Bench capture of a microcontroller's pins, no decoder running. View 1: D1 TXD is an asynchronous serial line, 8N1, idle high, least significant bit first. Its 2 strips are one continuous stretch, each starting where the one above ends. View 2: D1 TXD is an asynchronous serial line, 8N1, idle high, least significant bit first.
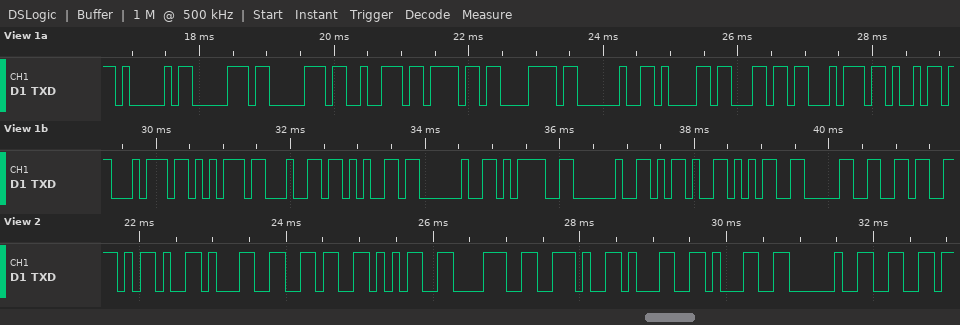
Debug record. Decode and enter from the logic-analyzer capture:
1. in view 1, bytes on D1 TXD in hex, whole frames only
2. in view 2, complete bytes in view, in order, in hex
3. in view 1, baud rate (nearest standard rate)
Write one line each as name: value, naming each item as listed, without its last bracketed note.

in view 1, bytes on D1 TXD in hex, whole frames only: 0x41 0x70 0x70 0x72 0x6F 0x78 0x20 0x61 0x6C 0x74 0x69 0x74 0x75 0x64 0x65 0x20 0x3D 0x20 0x2D 0x35 0x30 0x36
in view 2, complete bytes in view, in order, in hex: 2D 31 36 35 38 2E 31 31 20 66
in view 1, baud rate: 9600 baud
